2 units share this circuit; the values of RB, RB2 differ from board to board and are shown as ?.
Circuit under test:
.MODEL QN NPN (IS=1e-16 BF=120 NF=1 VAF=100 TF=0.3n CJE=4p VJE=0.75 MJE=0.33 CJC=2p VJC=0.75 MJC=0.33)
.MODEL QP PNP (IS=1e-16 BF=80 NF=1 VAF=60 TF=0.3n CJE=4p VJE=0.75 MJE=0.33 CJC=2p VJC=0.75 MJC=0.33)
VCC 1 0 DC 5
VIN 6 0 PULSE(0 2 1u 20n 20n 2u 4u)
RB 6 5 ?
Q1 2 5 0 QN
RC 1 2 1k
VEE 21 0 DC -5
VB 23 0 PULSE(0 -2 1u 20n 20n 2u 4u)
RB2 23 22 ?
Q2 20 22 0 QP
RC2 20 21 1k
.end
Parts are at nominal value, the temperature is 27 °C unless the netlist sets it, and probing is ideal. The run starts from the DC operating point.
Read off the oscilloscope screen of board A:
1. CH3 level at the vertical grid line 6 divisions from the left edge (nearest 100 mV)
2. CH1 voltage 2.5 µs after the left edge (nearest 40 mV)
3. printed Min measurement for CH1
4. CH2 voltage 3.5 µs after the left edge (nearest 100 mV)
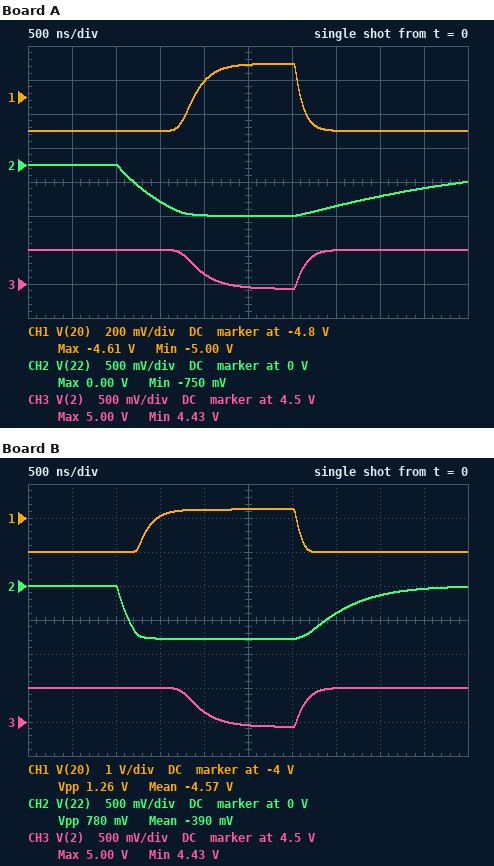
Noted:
4.4 V
-4.60 V
-5.00 V
-600 mV
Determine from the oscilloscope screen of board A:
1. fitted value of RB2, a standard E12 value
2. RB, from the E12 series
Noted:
270 kΩ
270 kΩ
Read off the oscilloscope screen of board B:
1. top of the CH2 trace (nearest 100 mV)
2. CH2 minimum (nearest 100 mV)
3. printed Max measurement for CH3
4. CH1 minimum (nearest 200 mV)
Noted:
0 V
-800 mV
5.00 V
-5.0 V
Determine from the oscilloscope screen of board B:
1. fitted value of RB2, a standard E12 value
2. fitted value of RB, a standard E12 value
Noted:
82 kΩ
270 kΩ
